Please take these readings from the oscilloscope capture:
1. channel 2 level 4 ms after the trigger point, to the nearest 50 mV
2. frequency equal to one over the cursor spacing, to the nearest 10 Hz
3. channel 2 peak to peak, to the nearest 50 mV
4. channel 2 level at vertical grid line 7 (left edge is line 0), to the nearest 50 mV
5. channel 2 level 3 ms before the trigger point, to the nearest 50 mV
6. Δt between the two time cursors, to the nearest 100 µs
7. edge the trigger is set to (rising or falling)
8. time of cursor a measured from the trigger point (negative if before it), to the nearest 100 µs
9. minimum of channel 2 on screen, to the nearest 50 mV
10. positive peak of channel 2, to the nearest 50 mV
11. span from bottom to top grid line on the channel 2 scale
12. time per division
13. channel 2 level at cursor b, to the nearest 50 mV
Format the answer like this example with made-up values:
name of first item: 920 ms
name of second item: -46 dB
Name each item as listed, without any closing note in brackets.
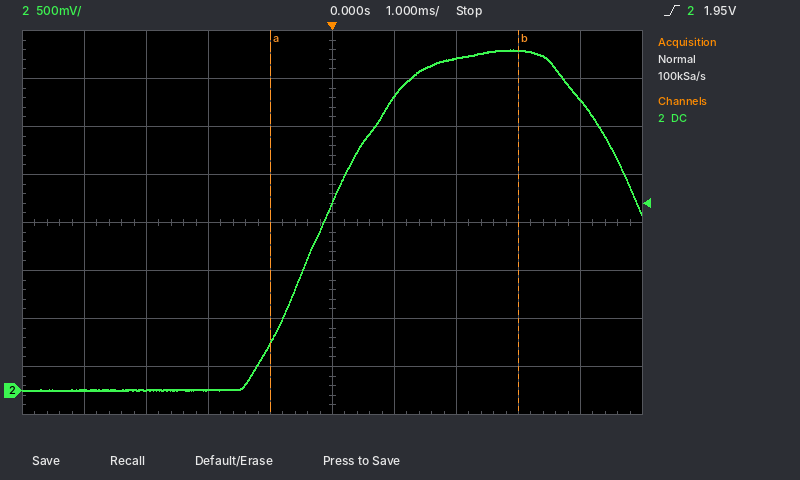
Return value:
channel 2 level 4 ms after the trigger point, to the nearest 50 mV: 3.05 V
frequency equal to one over the cursor spacing, to the nearest 10 Hz: 250 Hz
channel 2 peak to peak, to the nearest 50 mV: 3.55 V
channel 2 level at vertical grid line 7 (left edge is line 0), to the nearest 50 mV: 3.45 V
channel 2 level 3 ms before the trigger point, to the nearest 50 mV: 0 mV
Δt between the two time cursors, to the nearest 100 µs: 4.0 ms
edge the trigger is set to: rising
time of cursor a measured from the trigger point (negative if before it), to the nearest 100 µs: -1.0 ms
minimum of channel 2 on screen, to the nearest 50 mV: 0 mV
positive peak of channel 2, to the nearest 50 mV: 3.55 V
span from bottom to top grid line on the channel 2 scale: 4 V
time per division: 1 ms
channel 2 level at cursor b, to the nearest 50 mV: 3.55 V
